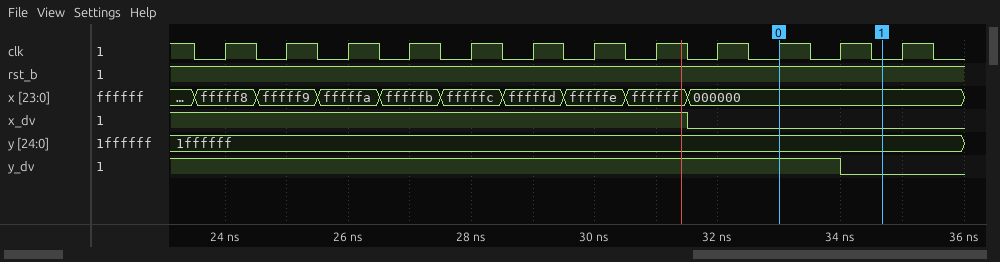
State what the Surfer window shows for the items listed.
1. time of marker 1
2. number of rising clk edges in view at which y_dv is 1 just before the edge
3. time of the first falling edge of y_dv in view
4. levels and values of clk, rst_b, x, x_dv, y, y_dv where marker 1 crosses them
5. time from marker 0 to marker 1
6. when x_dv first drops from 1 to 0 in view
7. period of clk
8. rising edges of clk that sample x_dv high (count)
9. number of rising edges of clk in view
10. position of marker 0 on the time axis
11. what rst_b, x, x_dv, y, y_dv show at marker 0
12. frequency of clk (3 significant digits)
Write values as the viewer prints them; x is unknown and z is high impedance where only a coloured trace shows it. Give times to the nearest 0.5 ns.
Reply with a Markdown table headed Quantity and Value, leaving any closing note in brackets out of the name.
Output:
| Quantity | Value |
|---|---|
| time of marker 1 | 34.5 ns |
| number of rising clk edges in view at which y_dv is 1 just before the edge | 11 |
| time of the first falling edge of y_dv in view | 34 ns |
| levels and values of clk, rst_b, x, x_dv, y, y_dv where marker 1 crosses them | clk=0, rst_b=1, x=000000, x_dv=0, y=1ffffff, y_dv=0 |
| time from marker 0 to marker 1 | 1.5 ns |
| when x_dv first drops from 1 to 0 in view | 31.5 ns |
| period of clk | 1 ns |
| rising edges of clk that sample x_dv high | 8 |
| number of rising edges of clk in view | 12 |
| position of marker 0 on the time axis | 33 ns |
| what rst_b, x, x_dv, y, y_dv show at marker 0 | rst_b=1, x=000000, x_dv=0, y=1ffffff, y_dv=1 |
| frequency of clk | 1.00 GHz |
